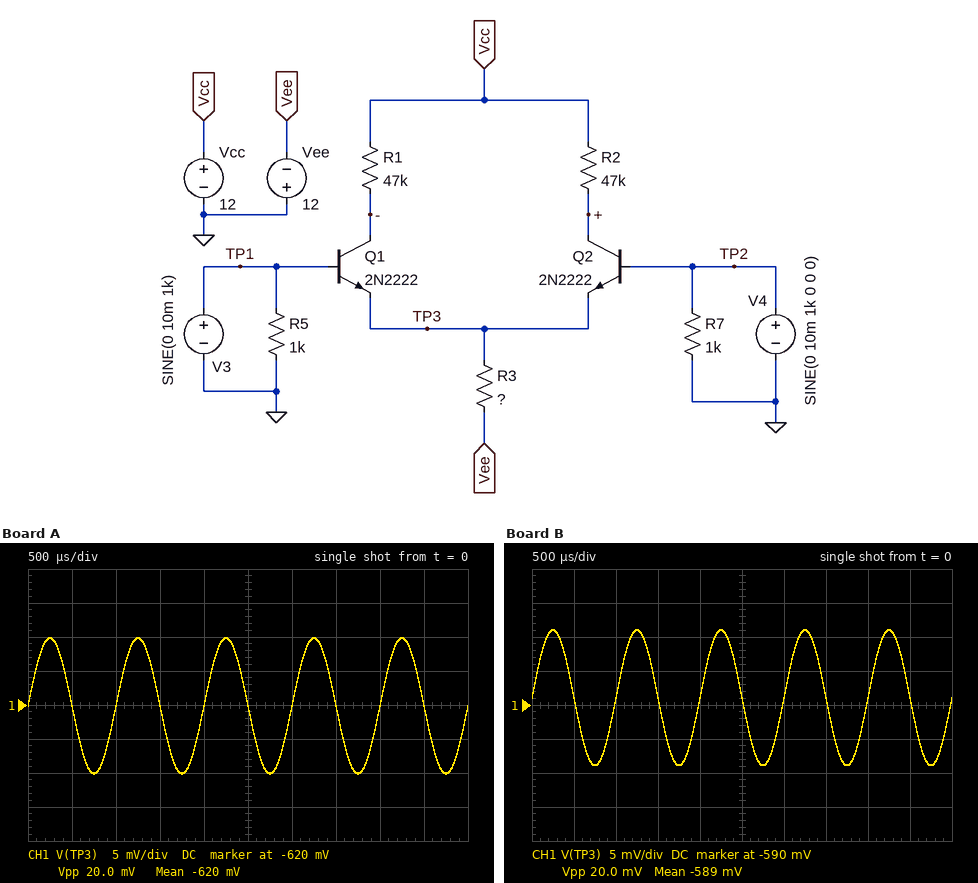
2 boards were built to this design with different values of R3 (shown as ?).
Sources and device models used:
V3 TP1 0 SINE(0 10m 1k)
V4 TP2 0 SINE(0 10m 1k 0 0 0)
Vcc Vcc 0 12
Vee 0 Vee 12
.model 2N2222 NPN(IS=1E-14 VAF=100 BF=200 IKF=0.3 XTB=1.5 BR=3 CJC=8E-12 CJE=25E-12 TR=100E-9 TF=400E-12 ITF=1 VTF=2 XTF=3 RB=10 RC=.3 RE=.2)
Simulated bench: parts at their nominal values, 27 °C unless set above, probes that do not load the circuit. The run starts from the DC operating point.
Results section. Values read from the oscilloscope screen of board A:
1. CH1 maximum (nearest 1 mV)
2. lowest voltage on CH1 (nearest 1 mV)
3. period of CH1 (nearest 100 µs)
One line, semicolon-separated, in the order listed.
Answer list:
-610 mV; -630 mV; 1.0 ms
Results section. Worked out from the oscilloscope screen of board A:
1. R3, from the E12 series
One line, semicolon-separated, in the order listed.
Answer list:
22 kΩ
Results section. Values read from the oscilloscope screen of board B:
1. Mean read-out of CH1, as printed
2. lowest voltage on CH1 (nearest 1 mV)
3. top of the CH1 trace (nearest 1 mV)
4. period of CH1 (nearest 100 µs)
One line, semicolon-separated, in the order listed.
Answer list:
-589 mV; -599 mV; -579 mV; 1.0 ms
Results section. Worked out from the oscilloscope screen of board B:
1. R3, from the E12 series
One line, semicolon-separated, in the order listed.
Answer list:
68 kΩ
